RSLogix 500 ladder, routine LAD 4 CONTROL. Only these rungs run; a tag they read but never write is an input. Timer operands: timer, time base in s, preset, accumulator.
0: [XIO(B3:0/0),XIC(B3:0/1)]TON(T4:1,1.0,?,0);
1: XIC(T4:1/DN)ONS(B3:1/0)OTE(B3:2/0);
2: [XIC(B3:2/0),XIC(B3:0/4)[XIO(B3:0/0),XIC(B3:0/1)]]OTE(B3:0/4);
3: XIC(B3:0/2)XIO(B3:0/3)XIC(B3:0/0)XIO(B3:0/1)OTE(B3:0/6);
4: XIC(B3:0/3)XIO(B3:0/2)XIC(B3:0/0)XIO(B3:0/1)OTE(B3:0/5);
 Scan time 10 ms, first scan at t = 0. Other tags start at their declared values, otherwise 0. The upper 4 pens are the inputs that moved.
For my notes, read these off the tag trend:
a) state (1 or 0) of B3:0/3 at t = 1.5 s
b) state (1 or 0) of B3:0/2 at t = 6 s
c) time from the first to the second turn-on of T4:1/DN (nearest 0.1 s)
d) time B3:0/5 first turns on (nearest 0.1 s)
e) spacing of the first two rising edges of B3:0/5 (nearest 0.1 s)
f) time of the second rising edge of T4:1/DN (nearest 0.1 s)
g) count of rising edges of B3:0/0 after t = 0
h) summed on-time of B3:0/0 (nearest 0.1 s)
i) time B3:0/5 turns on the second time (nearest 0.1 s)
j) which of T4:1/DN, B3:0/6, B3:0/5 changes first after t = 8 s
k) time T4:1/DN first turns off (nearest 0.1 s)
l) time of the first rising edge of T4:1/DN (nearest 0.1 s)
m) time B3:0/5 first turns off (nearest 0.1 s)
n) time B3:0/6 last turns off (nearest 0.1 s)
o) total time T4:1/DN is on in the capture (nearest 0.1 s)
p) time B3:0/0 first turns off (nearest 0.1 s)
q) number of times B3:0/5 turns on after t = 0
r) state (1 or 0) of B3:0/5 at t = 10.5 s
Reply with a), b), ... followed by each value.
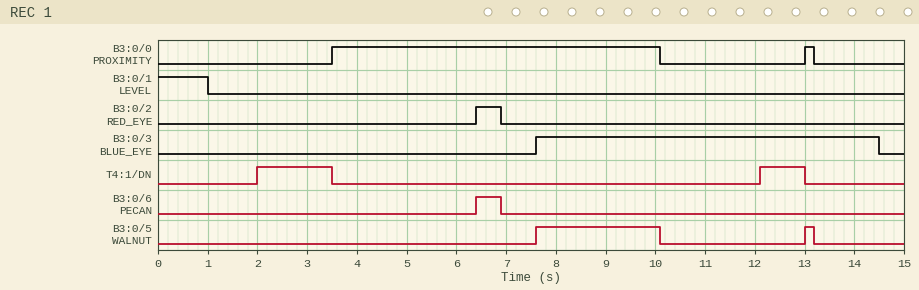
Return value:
a) 0
b) 0
c) 10.1 s
d) 7.6 s
e) 5.4 s
f) 12.1 s
g) 2
h) 6.8 s
i) 13.0 s
j) B3:0/5
k) 3.5 s
l) 2.0 s
m) 10.1 s
n) 6.9 s
o) 2.4 s
p) 10.1 s
q) 2
r) 0
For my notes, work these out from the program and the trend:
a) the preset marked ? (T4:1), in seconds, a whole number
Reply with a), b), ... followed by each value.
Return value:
a) 2 s
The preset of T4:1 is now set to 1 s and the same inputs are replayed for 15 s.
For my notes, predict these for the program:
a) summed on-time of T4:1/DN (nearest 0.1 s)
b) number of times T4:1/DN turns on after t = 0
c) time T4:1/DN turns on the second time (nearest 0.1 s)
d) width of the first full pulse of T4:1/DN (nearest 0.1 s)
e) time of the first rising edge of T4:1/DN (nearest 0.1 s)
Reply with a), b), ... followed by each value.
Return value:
a) 5.2 s
b) 3
c) 11.1 s
d) 2.5 s
e) 1.0 s
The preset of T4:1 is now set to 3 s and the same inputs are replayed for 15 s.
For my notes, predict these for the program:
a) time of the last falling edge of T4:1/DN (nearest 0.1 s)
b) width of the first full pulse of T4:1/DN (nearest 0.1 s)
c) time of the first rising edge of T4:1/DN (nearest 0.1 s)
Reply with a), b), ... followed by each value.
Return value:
a) 3.5 s
b) 0.5 s
c) 3.0 s
